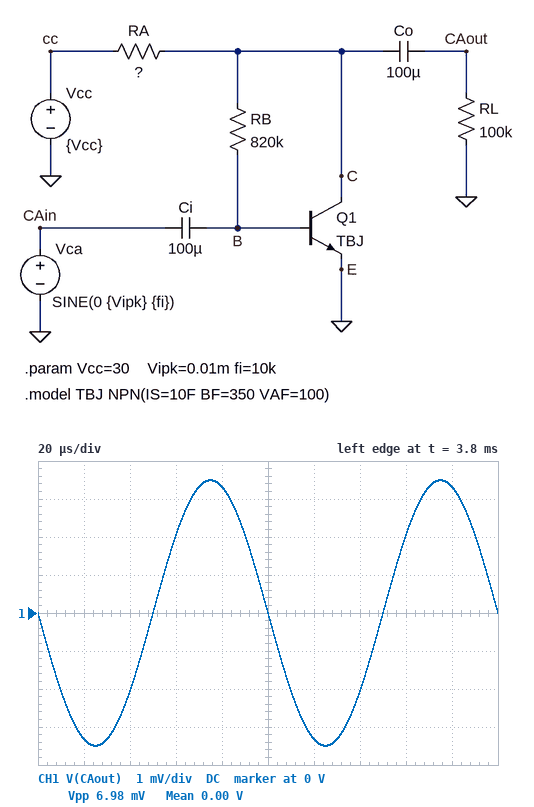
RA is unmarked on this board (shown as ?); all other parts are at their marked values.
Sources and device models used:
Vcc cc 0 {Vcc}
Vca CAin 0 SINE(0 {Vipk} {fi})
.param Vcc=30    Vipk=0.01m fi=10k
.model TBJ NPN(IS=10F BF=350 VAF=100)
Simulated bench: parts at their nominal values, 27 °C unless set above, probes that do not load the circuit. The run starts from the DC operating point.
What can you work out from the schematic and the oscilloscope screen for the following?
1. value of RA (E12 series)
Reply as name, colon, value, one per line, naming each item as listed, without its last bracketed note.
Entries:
value of RA: 1 kΩ
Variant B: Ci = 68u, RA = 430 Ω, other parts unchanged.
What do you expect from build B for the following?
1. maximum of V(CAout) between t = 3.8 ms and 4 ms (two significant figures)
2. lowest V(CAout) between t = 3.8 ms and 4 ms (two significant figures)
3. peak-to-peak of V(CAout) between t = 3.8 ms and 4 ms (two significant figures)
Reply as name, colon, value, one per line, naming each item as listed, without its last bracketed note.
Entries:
maximum of V(CAout) between t = 3.8 ms and 4 ms: 2.0 mV
lowest V(CAout) between t = 3.8 ms and 4 ms: -2.0 mV
peak-to-peak of V(CAout) between t = 3.8 ms and 4 ms: 4.0 mV
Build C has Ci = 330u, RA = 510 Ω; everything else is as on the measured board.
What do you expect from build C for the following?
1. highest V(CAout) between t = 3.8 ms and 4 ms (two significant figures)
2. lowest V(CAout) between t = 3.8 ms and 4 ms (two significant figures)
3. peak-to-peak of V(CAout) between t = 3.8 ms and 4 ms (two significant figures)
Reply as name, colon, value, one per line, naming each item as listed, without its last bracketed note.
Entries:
highest V(CAout) between t = 3.8 ms and 4 ms: 2.3 mV
lowest V(CAout) between t = 3.8 ms and 4 ms: -2.3 mV
peak-to-peak of V(CAout) between t = 3.8 ms and 4 ms: 4.5 mV
